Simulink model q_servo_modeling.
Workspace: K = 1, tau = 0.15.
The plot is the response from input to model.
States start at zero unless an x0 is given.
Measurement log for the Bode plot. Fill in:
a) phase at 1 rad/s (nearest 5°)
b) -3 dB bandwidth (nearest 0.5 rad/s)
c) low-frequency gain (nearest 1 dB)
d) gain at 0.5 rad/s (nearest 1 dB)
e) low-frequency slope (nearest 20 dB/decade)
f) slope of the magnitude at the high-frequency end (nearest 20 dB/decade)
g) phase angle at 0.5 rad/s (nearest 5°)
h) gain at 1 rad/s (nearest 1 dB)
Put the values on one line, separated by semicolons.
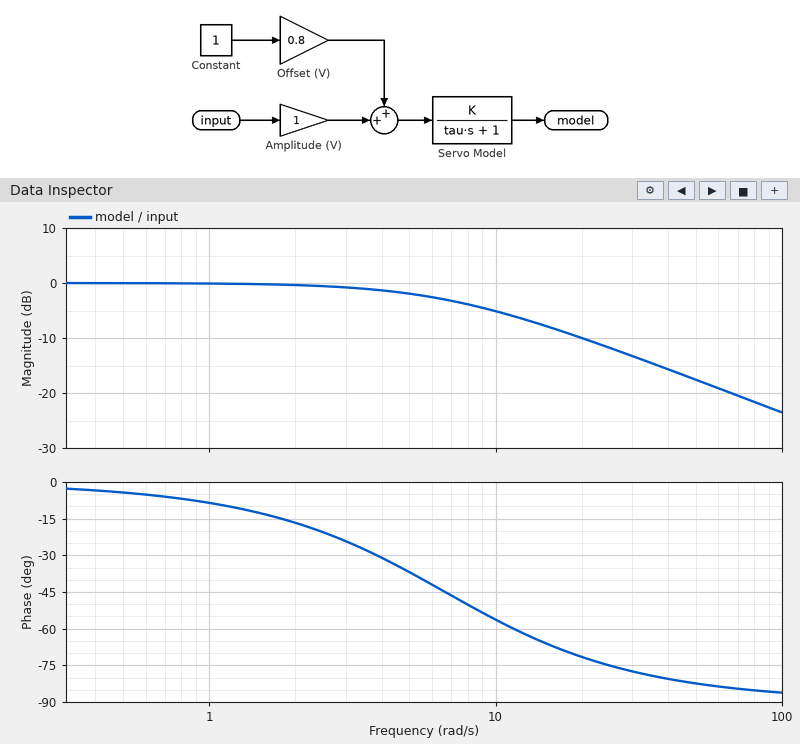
-10°; 6.5 rad/s; 0 dB; 0 dB; 0 dB/decade; -20 dB/decade; -5°; 0 dB
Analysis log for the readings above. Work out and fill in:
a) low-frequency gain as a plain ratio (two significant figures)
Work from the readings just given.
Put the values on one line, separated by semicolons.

1.0
